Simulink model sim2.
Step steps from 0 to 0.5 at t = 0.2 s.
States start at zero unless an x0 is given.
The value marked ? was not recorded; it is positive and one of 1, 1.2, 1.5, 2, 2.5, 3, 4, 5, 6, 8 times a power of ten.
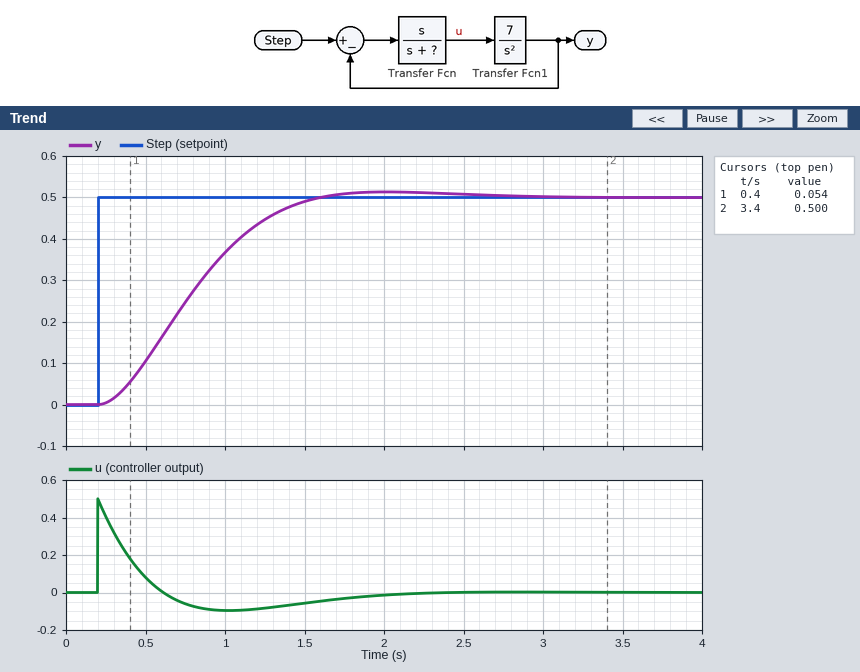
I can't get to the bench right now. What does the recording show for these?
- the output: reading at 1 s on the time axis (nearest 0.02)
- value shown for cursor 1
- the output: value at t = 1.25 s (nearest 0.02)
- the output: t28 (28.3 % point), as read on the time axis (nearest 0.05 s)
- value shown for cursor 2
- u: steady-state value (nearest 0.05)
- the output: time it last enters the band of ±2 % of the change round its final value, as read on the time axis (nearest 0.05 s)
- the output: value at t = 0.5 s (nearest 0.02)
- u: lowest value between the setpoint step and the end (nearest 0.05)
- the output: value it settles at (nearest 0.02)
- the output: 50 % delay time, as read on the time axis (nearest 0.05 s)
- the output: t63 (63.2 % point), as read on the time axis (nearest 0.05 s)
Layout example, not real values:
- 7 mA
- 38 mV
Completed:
- 0.36
- 0.054
- 0.44
- 0.55 s
- 0.500
- 0.00
- 2.35 s
- 0.10
- -0.10
- 0.50
- 0.75 s
- 0.90 s
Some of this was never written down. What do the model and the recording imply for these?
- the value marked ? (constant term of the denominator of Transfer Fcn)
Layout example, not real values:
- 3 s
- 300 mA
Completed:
- 4
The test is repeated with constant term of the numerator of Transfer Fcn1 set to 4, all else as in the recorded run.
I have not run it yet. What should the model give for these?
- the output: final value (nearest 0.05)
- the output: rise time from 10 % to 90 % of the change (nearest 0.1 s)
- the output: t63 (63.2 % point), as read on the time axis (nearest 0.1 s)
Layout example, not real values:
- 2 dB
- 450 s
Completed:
- 0.50
- 1.7 s
- 1.3 s
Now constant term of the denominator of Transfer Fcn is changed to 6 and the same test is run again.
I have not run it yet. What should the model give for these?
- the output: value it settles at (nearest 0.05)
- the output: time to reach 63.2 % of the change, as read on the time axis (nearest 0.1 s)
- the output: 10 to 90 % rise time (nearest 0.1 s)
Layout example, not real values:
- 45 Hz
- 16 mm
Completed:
- 0.50
- 1.1 s
- 1.5 s
